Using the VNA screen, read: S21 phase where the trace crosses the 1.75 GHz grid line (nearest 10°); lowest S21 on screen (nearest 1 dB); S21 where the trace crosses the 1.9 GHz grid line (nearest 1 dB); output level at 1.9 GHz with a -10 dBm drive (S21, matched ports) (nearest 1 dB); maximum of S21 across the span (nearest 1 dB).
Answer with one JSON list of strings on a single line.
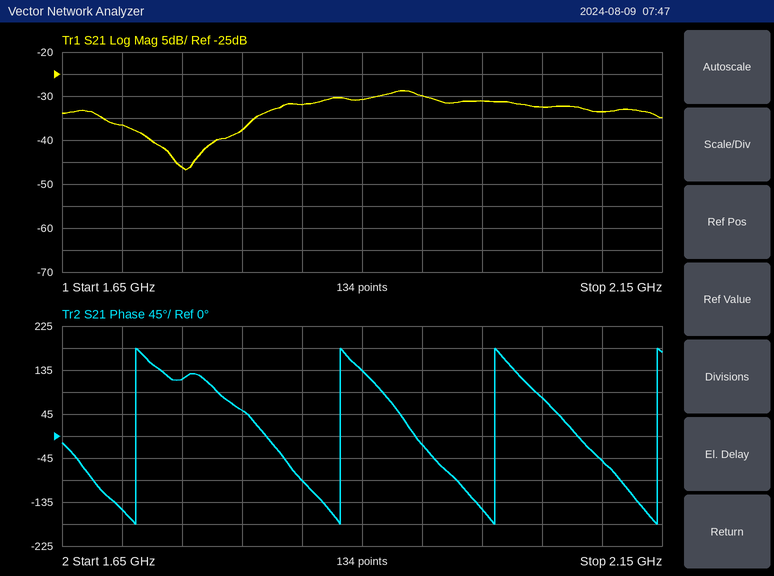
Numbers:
["120°", "-47 dB", "-31 dB", "-41 dBm", "-29 dB"]
